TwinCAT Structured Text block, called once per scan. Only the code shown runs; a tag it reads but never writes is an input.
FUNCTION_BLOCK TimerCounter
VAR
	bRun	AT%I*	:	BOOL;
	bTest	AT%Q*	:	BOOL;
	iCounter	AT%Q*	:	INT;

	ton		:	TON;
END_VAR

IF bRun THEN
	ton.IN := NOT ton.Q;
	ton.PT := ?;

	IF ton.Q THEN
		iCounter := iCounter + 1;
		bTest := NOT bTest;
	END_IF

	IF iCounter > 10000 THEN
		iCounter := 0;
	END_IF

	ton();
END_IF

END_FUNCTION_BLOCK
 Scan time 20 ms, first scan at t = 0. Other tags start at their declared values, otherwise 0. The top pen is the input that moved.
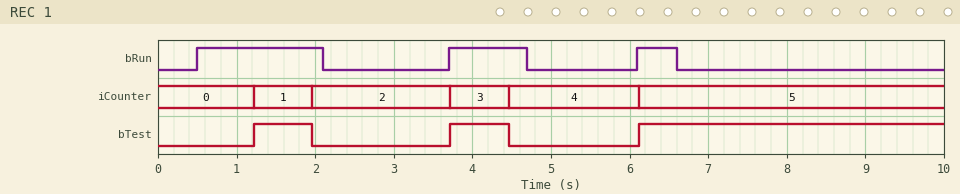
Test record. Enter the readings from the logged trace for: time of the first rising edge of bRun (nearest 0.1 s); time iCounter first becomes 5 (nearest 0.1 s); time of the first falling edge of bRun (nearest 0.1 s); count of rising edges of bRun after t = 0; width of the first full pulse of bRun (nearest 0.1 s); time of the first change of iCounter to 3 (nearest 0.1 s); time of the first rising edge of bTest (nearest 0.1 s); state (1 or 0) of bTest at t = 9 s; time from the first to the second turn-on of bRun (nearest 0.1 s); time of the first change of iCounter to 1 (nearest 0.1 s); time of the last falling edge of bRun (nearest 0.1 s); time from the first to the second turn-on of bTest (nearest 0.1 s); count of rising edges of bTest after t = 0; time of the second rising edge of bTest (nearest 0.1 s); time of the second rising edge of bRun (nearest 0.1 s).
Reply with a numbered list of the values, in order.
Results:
1. 0.5 s
2. 6.1 s
3. 2.1 s
4. 3
5. 1.6 s
6. 3.7 s
7. 1.2 s
8. 1
9. 3.2 s
10. 1.2 s
11. 6.6 s
12. 2.5 s
13. 3
14. 3.7 s
15. 3.7 s
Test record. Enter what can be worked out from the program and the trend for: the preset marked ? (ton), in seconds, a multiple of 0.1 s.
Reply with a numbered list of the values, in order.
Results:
1. 0.7 s
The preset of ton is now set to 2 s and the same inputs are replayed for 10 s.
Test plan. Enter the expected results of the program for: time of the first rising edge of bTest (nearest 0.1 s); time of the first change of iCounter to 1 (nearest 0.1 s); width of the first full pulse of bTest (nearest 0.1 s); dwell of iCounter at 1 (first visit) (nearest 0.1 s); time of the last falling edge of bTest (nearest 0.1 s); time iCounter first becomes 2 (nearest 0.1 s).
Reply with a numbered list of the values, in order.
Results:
1. 3.7 s
2. 3.7 s
3. 2.4 s
4. 2.4 s
5. 6.1 s
6. 6.1 s
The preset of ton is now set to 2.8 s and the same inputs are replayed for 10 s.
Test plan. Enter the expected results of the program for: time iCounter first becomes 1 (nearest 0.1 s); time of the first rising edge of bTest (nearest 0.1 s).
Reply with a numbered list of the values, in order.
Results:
1. 3.7 s
2. 3.7 s
